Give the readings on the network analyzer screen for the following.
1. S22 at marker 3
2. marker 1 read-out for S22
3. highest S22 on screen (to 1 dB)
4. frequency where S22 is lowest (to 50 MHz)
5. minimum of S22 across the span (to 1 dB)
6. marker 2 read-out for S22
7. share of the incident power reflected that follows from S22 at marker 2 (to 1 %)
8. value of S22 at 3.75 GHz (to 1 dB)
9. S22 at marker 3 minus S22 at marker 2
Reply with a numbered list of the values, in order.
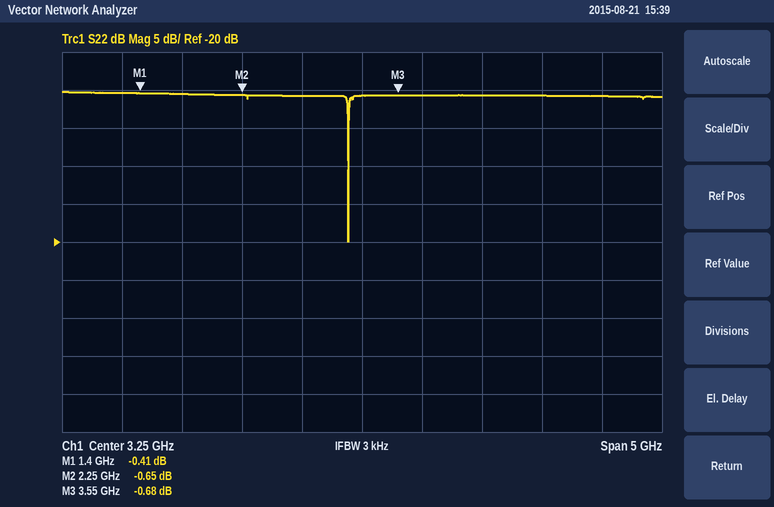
1. -0.68 dB
2. -0.41 dB
3. 0 dB
4. 3.15 GHz
5. -20 dB
6. -0.65 dB
7. 86 %
8. -1 dB
9. -0.03 dB
